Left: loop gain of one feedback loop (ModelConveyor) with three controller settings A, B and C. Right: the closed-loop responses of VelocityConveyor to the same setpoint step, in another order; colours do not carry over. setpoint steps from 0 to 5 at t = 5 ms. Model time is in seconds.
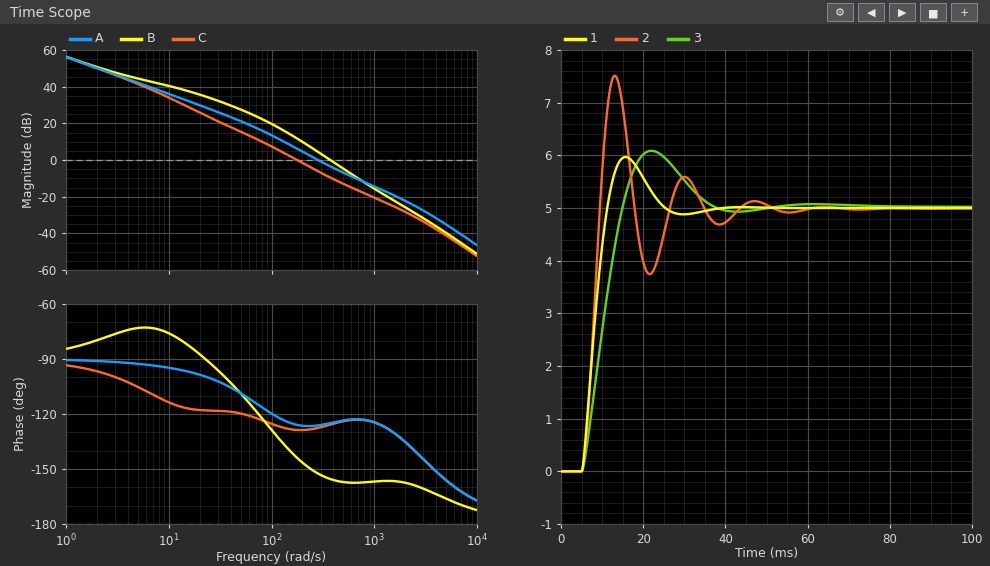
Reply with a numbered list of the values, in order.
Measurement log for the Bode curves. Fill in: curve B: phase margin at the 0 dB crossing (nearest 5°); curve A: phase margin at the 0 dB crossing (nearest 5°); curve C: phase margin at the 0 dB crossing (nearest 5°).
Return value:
1. 25°
2. 55°
3. 50°
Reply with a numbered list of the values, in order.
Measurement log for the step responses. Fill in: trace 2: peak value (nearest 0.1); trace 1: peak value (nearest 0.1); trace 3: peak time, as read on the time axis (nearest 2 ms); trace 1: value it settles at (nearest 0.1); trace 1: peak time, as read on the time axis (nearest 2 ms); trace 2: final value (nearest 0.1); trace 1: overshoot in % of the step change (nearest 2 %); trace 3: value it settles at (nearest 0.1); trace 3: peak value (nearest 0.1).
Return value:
1. 7.5
2. 6.0
3. 22 ms
4. 5.0
5. 16 ms
6. 5.0
7. 20 %
8. 5.0
9. 6.1
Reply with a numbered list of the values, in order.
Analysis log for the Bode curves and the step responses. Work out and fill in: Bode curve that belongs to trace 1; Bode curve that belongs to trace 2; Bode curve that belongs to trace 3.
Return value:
1. A
2. B
3. C
